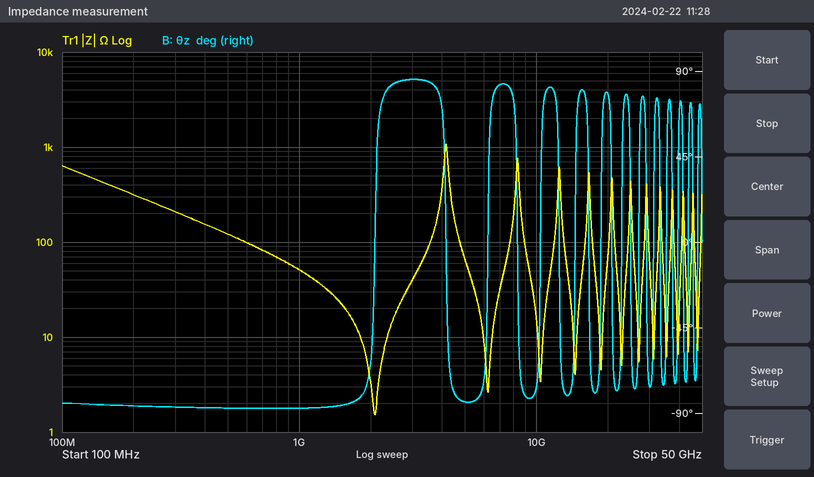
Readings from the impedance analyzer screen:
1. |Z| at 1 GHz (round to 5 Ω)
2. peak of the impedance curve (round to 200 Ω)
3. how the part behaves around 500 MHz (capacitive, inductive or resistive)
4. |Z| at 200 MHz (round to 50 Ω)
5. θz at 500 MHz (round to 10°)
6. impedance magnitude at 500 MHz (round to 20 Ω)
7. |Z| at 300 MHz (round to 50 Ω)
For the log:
50 Ω
1.0 kΩ
capacitive
300 Ω
-90°
120 Ω
200 Ω
